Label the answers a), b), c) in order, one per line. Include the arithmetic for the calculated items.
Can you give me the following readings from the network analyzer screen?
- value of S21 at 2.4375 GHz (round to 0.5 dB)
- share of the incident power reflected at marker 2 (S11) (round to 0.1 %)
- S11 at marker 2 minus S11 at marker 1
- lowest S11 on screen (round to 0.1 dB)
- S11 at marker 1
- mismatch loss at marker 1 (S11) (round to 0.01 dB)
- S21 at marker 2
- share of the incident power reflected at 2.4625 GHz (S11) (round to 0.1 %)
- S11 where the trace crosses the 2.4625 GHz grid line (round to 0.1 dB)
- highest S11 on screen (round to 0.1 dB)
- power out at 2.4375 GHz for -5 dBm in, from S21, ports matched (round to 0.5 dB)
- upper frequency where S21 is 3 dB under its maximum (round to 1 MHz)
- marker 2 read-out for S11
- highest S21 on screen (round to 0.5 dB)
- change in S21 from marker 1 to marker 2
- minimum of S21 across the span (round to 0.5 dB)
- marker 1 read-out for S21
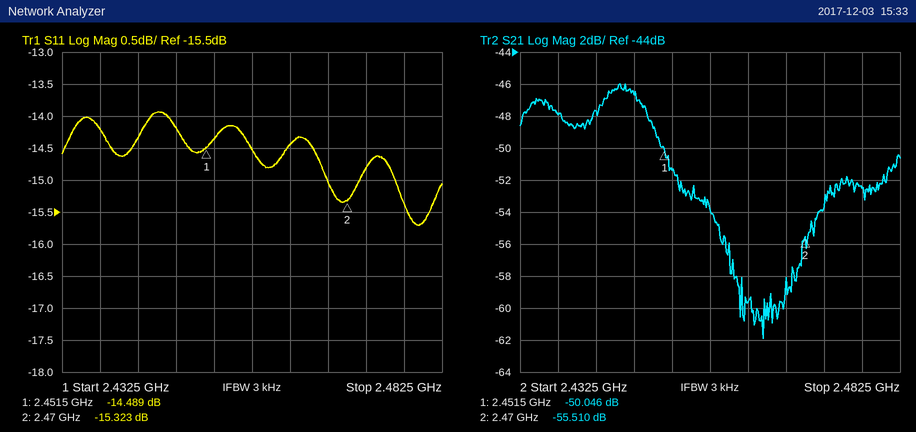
a) -48.0 dB
b) 10^(-15.323/10) ≈ 2.9 %
c) -15.323 − (-14.489) = -0.834 dB
d) -15.7 dB
e) -14.489 dB
f) −10 log10(1 − 10^(-14.489/10)) ≈ 0.16 dB
g) -55.510 dB
h) 10^(-14.4/10) ≈ 3.6 %
i) -14.4 dB
j) -13.9 dB
k) -5 dBm + (-48.0 dB) = -53.0 dBm
l) 2.450 GHz
m) -15.323 dB
n) -46.0 dB
o) -55.51 − (-50.046) = -5.464 dB
p) -62.0 dB
q) -50.046 dB
